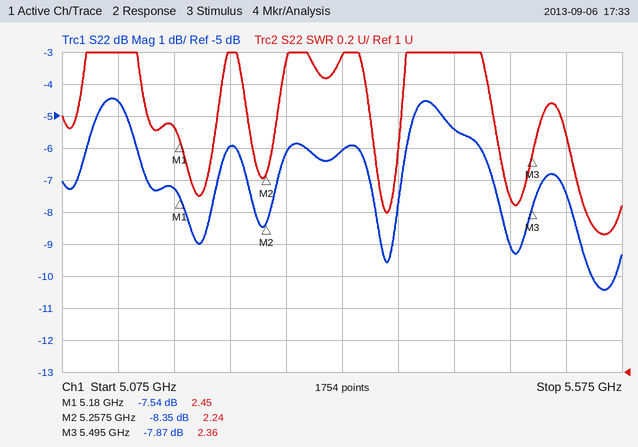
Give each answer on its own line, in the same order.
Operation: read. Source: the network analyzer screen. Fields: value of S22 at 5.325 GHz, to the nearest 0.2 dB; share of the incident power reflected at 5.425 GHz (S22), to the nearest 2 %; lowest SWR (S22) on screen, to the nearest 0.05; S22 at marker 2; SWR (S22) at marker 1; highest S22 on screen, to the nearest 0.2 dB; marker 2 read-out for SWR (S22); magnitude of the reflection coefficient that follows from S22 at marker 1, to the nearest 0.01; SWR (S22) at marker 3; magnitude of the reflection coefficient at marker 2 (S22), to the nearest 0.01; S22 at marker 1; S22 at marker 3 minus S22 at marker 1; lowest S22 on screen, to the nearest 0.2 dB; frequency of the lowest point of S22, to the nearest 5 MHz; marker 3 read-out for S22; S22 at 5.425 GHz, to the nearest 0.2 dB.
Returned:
-6.0 dB
28 %
1.85
-8.35 dB
2.45
-4.4 dB
2.24
0.42
2.36
0.38
-7.54 dB
-0.33 dB
-10.4 dB
5.560 GHz
-7.87 dB
-5.4 dB
